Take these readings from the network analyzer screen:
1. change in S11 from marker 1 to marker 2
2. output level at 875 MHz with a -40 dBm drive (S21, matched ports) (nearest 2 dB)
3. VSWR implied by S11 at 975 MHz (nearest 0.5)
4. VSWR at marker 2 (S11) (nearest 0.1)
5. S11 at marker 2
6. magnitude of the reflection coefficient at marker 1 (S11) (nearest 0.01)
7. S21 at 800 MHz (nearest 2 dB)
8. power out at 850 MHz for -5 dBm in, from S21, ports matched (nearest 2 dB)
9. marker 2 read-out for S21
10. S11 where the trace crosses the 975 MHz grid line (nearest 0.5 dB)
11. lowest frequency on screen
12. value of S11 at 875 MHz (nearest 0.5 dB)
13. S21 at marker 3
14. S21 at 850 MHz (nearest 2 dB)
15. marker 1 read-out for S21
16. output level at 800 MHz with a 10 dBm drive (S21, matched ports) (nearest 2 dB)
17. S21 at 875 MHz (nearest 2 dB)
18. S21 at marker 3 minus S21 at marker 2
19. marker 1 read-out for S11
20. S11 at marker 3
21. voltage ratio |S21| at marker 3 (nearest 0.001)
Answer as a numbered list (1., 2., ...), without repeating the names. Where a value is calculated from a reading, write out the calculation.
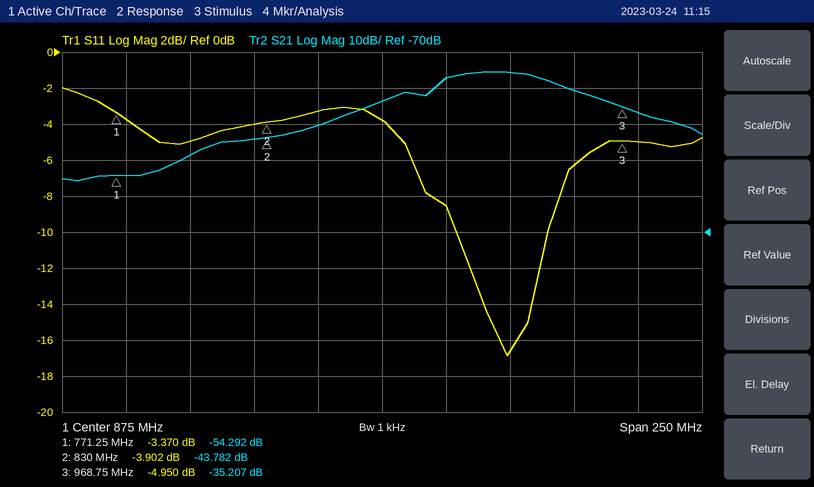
1. -3.902 − (-3.37) = -0.532 dB
2. -40 dBm + (-34 dB) = -74 dBm
3. |Γ| = 10^(-5/20) = 0.5623; VSWR = (1 + 0.5623)/(1 − 0.5623) ≈ 3.57, so 3.5 to the nearest 0.5
4. (1 + 0.6381)/(1 − 0.6381) ≈ 4.5
5. -3.902 dB
6. 10^(-3.37/20) ≈ 0.68
7. -48 dB
8. -5 dBm + (-40 dB) = -46 dBm
9. -43.782 dB
10. -5.0 dB
11. 750 MHz
12. -4.0 dB
13. -35.207 dB
14. -40 dB
15. -54.292 dB
16. 10 dBm + (-48 dB) = -38 dBm
17. -34 dB
18. -35.207 − (-43.782) = 8.575 dB
19. -3.370 dB
20. -4.950 dB
21. 10^(-35.207/20) ≈ 0.017
